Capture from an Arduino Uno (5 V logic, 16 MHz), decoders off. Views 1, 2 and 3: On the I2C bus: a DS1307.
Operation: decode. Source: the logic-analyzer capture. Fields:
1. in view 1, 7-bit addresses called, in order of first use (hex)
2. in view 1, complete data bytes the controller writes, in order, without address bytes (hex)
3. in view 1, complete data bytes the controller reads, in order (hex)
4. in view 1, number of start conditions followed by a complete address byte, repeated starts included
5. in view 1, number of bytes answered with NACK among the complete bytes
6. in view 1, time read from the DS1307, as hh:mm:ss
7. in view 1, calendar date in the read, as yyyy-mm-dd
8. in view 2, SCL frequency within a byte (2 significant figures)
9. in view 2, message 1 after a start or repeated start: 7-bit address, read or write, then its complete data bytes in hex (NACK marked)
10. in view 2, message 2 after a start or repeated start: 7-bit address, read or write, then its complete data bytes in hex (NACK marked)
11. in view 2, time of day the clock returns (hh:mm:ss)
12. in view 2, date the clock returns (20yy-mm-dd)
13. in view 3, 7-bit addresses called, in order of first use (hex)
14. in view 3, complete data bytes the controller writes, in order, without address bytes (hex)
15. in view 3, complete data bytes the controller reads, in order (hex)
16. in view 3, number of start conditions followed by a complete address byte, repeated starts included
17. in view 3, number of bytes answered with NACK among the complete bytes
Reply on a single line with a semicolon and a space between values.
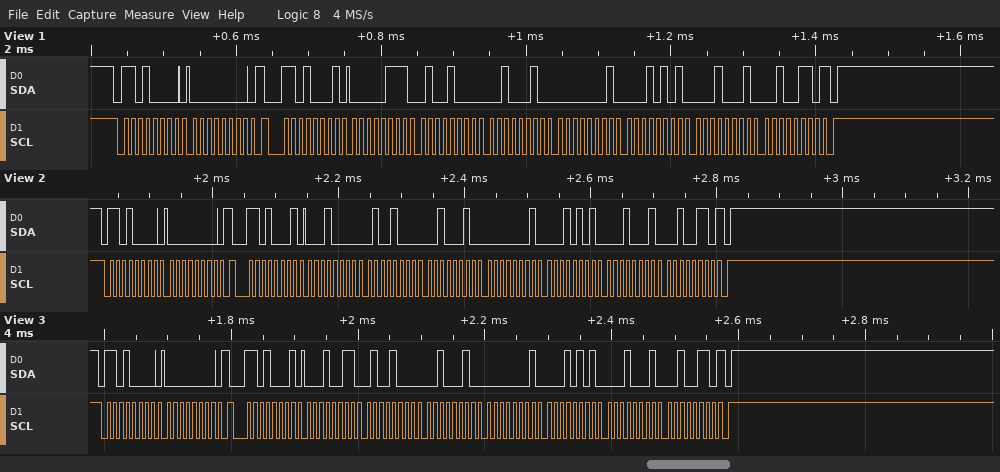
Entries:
0x68; 00; 07 48 22 01 15 11 26; 2; 1; 22:48:07; 2026-11-15; 100 kHz; 0x68 write: 00; 0x68 read: 10 48 22 01 15 11 26 NACK; 22:48:10; 2026-11-15; 0x68; 00; 13 48 22 01 15 11 26; 2; 1
